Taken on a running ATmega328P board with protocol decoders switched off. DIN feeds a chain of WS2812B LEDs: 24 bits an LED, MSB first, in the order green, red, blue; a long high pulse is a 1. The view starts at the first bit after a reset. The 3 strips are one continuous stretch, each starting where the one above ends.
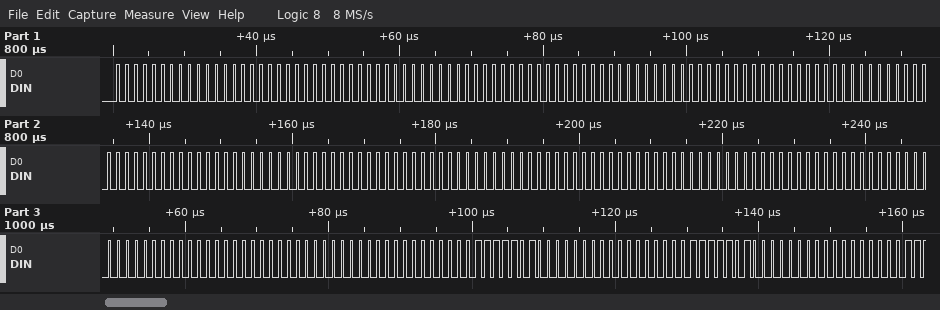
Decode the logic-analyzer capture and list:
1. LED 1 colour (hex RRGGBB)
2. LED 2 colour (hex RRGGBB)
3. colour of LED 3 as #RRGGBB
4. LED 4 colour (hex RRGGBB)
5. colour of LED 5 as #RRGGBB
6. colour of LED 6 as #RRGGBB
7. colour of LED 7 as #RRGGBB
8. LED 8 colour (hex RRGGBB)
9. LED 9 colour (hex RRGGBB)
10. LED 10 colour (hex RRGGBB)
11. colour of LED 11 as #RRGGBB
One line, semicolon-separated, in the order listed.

#000000; #000000; #000000; #000000; #000000; #000000; #000000; #000000; #000000; #FA0000; #FA0000
